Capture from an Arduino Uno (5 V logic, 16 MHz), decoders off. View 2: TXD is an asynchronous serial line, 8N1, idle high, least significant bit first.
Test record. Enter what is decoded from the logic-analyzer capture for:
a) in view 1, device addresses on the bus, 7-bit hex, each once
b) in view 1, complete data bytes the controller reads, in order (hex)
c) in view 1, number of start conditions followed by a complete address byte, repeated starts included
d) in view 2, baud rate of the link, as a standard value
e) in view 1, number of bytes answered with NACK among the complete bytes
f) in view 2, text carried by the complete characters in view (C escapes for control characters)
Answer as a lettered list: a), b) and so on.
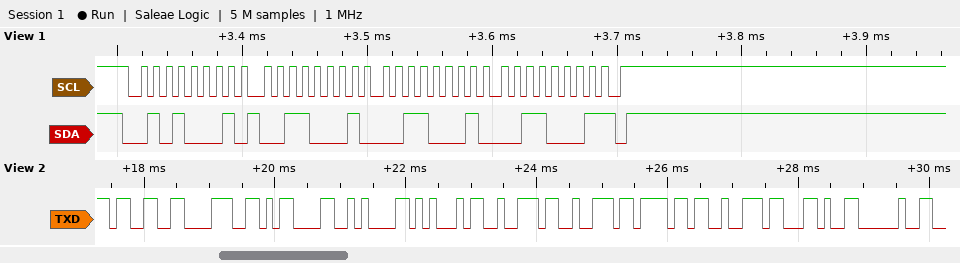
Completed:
a) 0x28
b) 31 31 31
c) 1
d) 9600 baud
e) 1
f) "38\r\nError, "
